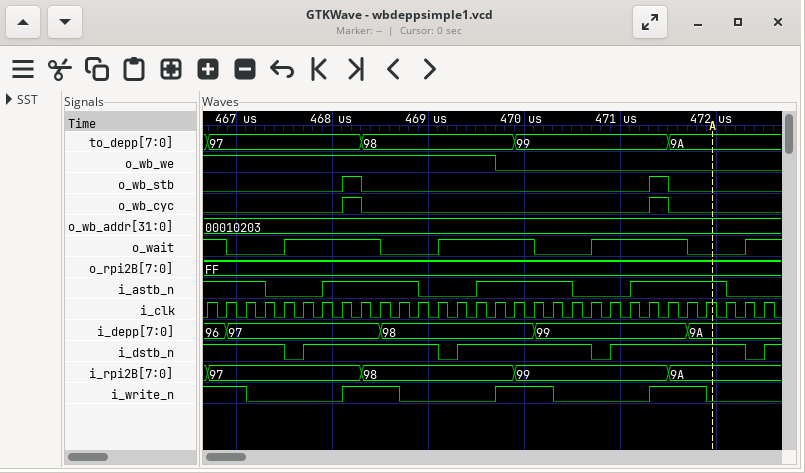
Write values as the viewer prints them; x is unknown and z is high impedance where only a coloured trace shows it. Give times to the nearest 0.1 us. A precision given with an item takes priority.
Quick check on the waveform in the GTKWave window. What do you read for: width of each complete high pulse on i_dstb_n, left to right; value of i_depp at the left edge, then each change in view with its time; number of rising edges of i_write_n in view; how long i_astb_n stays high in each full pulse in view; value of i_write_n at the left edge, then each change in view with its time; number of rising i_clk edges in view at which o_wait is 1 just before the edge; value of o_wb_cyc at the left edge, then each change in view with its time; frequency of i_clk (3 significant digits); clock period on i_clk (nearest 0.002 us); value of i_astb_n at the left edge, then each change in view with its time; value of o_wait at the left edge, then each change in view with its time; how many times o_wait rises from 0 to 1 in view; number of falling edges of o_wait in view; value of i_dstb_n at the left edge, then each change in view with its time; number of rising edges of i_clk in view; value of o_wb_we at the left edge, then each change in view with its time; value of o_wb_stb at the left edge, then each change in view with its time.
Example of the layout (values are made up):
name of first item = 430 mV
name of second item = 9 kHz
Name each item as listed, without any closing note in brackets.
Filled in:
width of each complete high pulse on i_dstb_n, left to right = 1.4 us, 1.4 us, 1.4 us
value of i_depp at the left edge, then each change in view with its time = 96, 97 at 466.9 us, 98 at 468.5 us, 99 at 470.1 us, 9A at 471.7 us
number of rising edges of i_write_n in view = 3
how long i_astb_n stays high in each full pulse in view = 1 us, 1 us, 1 us
value of i_write_n at the left edge, then each change in view with its time = 1, 0 at 467.1 us, 1 at 468.1 us, 0 at 468.7 us, 1 at 469.7 us, 0 at 470.3 us, 1 at 471.3 us, 0 at 471.9 us
number of rising i_clk edges in view at which o_wait is 1 just before the edge = 18
value of o_wb_cyc at the left edge, then each change in view with its time = 0, 1 at 468.1 us, 0 at 468.3 us, 1 at 471.3 us, 0 at 471.5 us
frequency of i_clk = 5.00 MHz
clock period on i_clk = 0.2 us
value of i_astb_n at the left edge, then each change in view with its time = 1, 0 at 467.3 us, 1 at 467.9 us, 0 at 468.9 us, 1 at 469.5 us, 0 at 470.5 us, 1 at 471.1 us, 0 at 472.1 us
value of o_wait at the left edge, then each change in view with its time = 1, 0 at 466.9 us, 1 at 467.5 us, 0 at 468.5 us, 1 at 469.1 us, 0 at 470.1 us, 1 at 470.7 us, 0 at 471.7 us, 1 at 472.3 us
how many times o_wait rises from 0 to 1 in view = 4
number of falling edges of o_wait in view = 4
value of i_dstb_n at the left edge, then each change in view with its time = 1, 0 at 467.5 us, 1 at 467.7 us, 0 at 469.1 us, 1 at 469.3 us, 0 at 470.7 us, 1 at 470.9 us, 0 at 472.3 us, 1 at 472.5 us
number of rising edges of i_clk in view = 30
value of o_wb_we at the left edge, then each change in view with its time = 1, 0 at 469.7 us
value of o_wb_stb at the left edge, then each change in view with its time = 0, 1 at 468.1 us, 0 at 468.3 us, 1 at 471.3 us, 0 at 471.5 us
